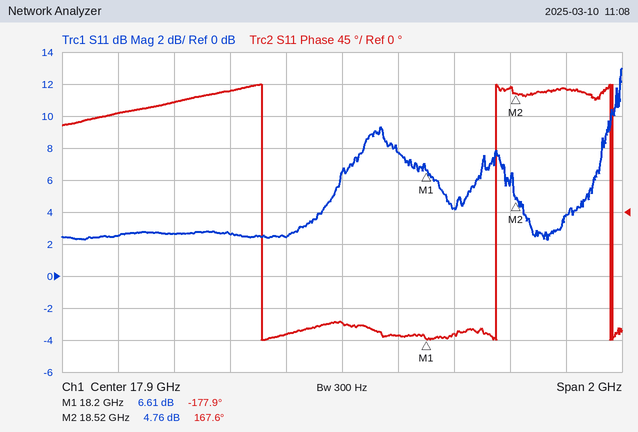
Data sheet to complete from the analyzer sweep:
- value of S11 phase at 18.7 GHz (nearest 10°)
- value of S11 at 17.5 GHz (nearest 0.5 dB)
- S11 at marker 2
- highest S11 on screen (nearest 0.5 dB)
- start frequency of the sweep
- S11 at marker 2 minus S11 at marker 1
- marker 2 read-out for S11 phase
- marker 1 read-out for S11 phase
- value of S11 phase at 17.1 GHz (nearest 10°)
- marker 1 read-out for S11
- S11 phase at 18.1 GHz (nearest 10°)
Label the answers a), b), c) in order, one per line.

a) 170°
b) 2.5 dB
c) 4.76 dB
d) 13.0 dB
e) 16.9 GHz
f) -1.85 dB
g) 167.6°
h) -177.9°
i) 140°
j) 6.61 dB
k) -170°
